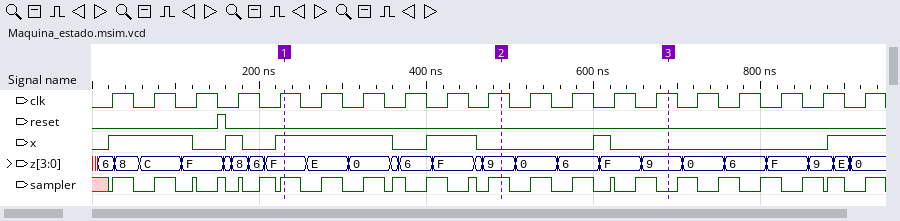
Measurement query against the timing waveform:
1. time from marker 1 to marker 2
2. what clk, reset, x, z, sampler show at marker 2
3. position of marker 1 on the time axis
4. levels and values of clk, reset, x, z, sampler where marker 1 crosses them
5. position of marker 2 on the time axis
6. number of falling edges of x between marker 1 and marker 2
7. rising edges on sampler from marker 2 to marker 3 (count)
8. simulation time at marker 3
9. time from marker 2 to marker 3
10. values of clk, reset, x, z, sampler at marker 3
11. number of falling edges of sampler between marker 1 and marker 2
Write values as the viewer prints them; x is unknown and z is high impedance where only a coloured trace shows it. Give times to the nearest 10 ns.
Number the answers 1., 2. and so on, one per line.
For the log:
1. 260 ns
2. clk=1, reset=0, x=0, z=9, sampler=1
3. 230 ns
4. clk=1, reset=0, x=1, z=F, sampler=1
5. 490 ns
6. 2
7. 4
8. 690 ns
9. 200 ns
10. clk=1, reset=0, x=0, z=9, sampler=0
11. 6
